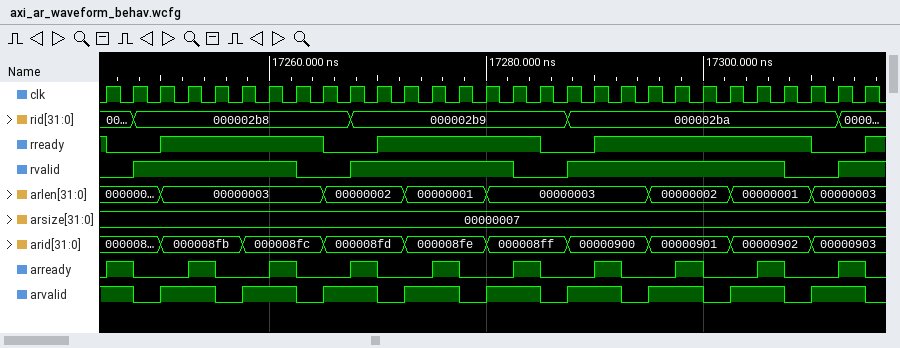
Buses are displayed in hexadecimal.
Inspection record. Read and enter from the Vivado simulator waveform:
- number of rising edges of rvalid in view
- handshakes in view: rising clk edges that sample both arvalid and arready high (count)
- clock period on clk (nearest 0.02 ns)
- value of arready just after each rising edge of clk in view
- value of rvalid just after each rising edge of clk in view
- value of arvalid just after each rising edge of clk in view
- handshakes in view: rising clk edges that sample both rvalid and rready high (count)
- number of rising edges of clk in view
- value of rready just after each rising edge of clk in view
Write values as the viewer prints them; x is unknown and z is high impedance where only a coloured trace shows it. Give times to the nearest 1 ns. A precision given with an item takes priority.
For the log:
4
10
2.5 ns
1 0 0 1 0 0 1 0 0 1 0 0 1 0 0 1 0 0 1 0 0 1 0 0 1 0 0 1 0
0 1 1 1 1 1 1 0 0 1 1 1 1 1 1 0 0 1 1 1 1 1 1 1 1 0 0 1 1
1 0 1 1 0 1 1 0 1 1 0 1 1 0 1 1 0 1 1 0 1 1 0 1 1 0 1 1 0
17
29
0 0 1 1 1 1 1 1 0 0 1 1 1 1 1 1 0 0 1 1 1 1 1 1 1 1 0 0 1
